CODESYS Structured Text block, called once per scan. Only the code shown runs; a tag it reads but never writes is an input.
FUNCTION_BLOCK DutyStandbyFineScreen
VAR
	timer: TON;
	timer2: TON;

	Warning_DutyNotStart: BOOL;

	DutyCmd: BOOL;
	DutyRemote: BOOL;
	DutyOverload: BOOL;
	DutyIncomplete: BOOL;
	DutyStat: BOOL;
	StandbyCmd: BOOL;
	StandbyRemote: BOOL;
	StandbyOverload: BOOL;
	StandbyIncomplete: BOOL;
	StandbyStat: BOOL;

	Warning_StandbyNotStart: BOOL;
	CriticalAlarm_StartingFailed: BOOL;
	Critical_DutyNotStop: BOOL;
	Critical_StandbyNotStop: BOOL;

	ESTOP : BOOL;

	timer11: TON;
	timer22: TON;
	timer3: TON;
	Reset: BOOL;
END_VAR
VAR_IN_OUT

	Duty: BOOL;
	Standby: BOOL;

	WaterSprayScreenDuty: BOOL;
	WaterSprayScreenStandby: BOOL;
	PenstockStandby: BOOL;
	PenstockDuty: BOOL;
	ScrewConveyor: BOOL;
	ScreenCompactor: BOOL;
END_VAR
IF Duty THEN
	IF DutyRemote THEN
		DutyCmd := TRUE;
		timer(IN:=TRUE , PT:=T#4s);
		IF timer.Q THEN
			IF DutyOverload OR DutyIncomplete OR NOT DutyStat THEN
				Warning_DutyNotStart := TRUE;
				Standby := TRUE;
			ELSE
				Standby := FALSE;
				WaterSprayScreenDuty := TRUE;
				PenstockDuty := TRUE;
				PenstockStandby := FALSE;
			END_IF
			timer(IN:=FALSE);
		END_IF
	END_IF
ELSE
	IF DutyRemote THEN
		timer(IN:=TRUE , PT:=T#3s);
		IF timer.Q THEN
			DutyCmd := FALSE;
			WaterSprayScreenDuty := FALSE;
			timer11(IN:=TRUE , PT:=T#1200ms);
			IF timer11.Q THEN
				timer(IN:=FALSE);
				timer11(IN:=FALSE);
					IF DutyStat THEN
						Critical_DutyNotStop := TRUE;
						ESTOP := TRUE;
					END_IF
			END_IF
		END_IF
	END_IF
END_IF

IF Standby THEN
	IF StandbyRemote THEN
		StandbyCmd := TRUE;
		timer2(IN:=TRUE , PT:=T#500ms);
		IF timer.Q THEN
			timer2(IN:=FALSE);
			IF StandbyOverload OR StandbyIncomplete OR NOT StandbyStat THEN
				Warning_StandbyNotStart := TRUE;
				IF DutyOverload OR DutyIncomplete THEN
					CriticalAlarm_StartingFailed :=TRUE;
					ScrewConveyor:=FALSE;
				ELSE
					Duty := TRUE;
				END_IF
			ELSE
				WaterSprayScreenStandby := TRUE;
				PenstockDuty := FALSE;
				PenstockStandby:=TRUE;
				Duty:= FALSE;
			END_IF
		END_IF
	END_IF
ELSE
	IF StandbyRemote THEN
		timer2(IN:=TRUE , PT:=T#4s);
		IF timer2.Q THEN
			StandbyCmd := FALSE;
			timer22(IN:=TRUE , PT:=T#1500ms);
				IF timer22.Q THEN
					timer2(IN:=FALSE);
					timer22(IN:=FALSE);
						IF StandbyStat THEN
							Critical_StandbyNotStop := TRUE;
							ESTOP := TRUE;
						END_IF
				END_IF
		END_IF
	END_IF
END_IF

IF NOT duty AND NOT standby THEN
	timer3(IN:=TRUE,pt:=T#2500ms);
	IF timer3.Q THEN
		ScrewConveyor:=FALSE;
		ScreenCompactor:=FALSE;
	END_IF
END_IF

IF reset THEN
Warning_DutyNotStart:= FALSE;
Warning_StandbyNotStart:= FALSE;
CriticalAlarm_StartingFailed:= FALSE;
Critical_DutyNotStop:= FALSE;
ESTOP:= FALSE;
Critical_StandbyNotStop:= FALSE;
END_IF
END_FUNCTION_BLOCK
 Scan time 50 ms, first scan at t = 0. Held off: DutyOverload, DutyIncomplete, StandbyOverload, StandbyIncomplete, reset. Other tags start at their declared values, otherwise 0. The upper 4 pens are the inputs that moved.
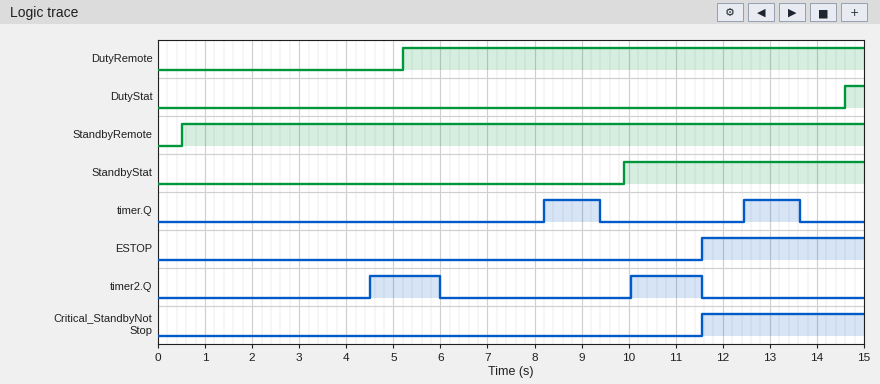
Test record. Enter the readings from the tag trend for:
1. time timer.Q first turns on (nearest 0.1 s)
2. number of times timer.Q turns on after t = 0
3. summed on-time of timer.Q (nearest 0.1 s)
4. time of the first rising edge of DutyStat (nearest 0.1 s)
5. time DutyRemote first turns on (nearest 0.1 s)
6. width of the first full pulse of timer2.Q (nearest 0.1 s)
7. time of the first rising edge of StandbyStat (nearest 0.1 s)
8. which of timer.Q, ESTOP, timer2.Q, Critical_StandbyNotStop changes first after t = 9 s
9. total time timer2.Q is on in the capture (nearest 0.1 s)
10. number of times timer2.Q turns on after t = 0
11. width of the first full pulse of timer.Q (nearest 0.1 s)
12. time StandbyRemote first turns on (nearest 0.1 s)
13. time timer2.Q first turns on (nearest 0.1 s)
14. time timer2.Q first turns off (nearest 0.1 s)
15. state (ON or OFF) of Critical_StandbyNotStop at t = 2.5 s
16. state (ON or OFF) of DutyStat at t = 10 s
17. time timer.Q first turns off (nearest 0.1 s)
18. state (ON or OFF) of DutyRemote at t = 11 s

8.2 s
2
2.4 s
14.6 s
5.2 s
1.5 s
9.9 s
timer.Q
3.0 s
2
1.2 s
0.5 s
4.5 s
6.0 s
OFF
OFF
9.4 s
ON
